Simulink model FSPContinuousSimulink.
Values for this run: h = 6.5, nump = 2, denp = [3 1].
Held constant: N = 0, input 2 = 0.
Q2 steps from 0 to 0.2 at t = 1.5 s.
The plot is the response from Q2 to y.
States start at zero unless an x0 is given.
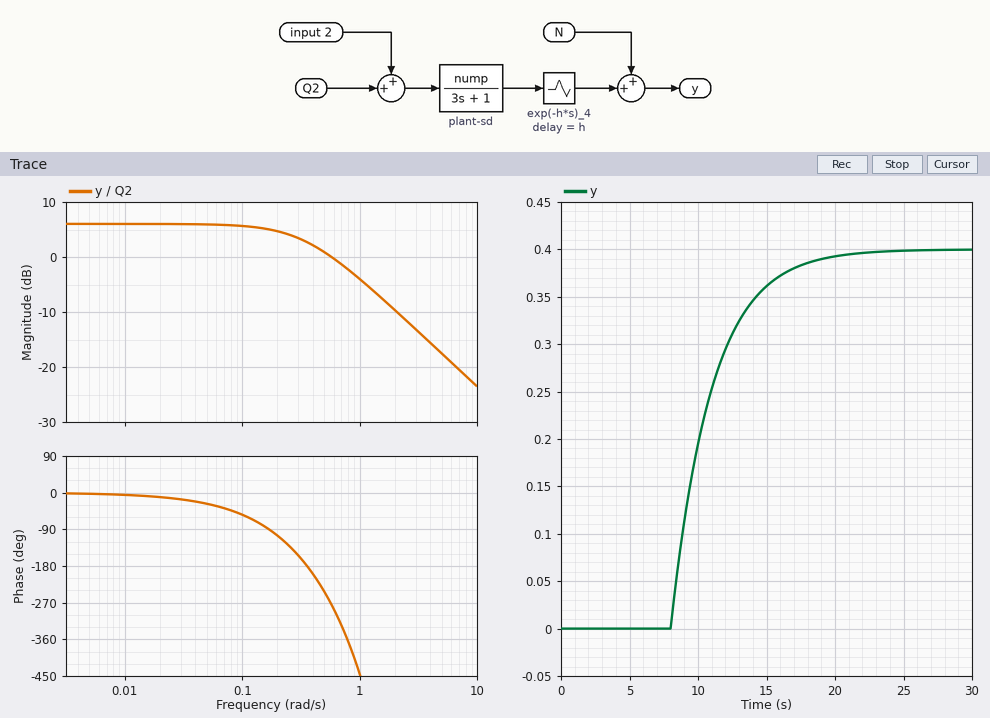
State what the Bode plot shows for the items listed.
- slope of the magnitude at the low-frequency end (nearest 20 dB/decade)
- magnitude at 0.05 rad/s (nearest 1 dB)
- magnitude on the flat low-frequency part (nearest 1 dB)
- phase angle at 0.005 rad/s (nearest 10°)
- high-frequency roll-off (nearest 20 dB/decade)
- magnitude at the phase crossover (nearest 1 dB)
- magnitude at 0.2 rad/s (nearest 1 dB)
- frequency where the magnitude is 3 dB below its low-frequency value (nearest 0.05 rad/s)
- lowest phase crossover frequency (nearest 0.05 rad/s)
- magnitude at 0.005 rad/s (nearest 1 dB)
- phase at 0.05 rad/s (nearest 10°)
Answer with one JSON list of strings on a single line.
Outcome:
["0 dB/decade", "6 dB", "6 dB", "0°", "-20 dB/decade", "3 dB", "5 dB", "0.35 rad/s", "0.35 rad/s", "6 dB", "-30°"]
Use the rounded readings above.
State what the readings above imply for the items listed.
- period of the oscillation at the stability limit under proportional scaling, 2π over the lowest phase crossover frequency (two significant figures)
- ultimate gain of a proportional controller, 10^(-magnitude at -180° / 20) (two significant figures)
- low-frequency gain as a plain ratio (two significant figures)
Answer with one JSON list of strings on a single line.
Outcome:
["18 s", "0.71", "2.0"]
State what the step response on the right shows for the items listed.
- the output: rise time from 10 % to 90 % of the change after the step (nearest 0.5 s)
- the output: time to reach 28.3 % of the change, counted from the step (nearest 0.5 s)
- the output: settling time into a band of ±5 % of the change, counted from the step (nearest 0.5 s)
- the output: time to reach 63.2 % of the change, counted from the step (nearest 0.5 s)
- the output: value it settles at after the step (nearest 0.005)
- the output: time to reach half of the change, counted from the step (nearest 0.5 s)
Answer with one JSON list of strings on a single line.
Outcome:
["6.5 s", "7.5 s", "15.5 s", "9.5 s", "0.400", "8.5 s"]
